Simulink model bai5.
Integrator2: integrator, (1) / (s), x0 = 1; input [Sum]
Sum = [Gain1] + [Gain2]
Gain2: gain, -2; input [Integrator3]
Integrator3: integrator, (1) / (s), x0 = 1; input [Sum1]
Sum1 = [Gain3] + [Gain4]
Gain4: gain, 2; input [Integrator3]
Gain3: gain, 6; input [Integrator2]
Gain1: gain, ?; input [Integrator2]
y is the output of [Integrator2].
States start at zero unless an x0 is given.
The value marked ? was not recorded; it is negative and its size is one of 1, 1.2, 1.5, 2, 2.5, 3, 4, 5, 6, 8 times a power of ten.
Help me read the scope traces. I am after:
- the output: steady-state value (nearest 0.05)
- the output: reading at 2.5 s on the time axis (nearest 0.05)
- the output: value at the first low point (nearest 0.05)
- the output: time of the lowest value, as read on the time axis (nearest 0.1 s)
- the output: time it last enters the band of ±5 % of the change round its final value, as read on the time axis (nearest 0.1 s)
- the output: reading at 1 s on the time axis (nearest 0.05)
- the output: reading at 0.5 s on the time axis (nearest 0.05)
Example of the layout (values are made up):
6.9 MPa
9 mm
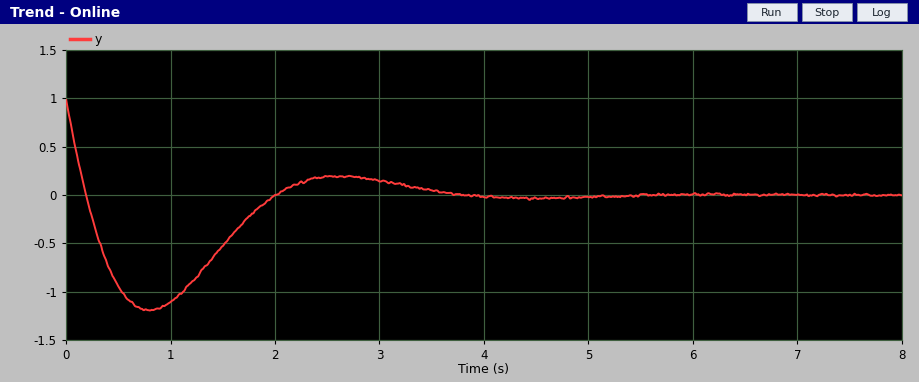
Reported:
0.00
0.20
-1.20
0.8 s
3.5 s
-1.10
-0.95
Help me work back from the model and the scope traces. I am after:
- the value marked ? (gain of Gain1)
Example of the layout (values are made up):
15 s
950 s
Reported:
-4
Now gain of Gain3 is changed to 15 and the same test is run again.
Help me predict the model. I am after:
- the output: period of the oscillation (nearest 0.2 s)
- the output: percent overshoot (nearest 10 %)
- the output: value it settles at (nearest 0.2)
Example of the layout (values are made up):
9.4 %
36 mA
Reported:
1.4 s
90 %
0.0
